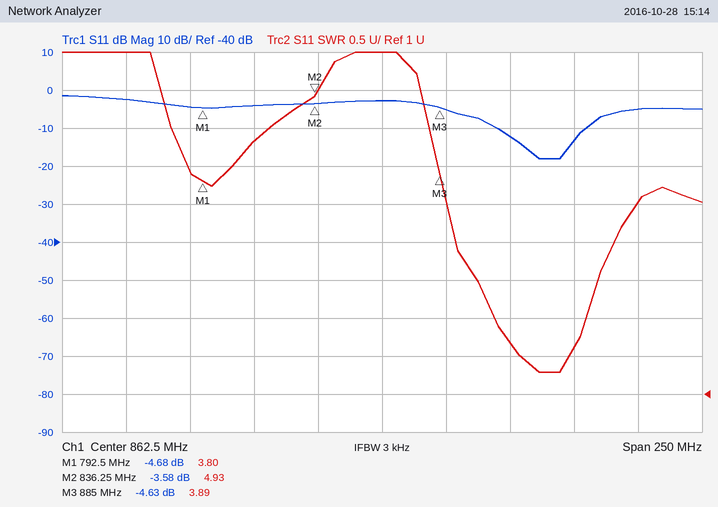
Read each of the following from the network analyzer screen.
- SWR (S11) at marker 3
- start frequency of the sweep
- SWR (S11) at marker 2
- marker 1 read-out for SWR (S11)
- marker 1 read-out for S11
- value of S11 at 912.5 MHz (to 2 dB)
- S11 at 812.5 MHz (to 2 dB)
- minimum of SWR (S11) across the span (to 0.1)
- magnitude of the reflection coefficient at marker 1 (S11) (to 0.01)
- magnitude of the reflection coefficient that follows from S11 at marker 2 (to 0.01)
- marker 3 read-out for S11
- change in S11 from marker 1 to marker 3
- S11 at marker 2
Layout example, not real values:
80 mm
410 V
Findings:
3.89
737.5 MHz
4.93
3.80
-4.68 dB
-12 dB
-4 dB
1.3
0.58
0.66
-4.63 dB
0.05 dB
-3.58 dB
